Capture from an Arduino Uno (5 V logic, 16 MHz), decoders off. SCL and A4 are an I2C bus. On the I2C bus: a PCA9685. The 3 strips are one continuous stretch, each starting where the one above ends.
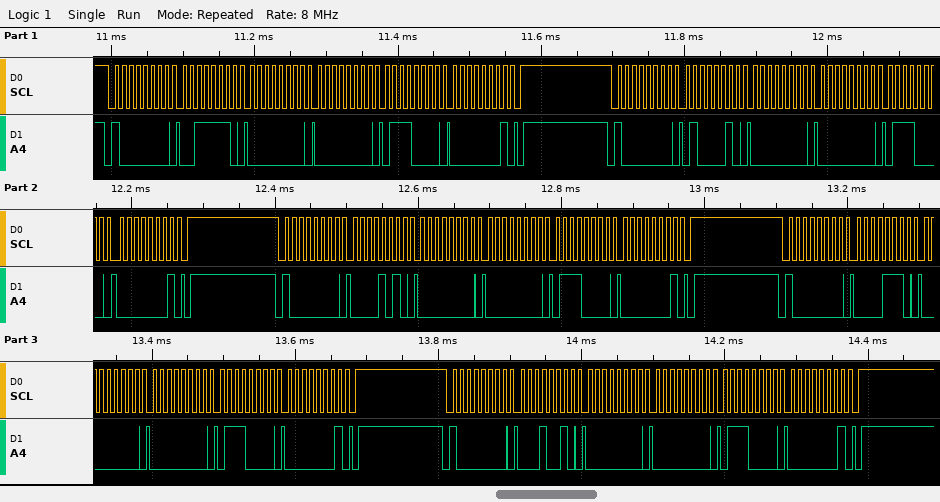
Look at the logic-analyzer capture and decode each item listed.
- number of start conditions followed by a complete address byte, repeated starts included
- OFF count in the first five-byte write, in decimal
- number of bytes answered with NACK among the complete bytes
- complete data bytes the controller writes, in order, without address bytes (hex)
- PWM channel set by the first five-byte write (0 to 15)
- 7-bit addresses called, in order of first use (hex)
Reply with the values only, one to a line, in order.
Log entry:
5
368
0
3E 00 00 70 01 42 00 00 70 01 0A 00 00 70 01 0E 00 00 70 01 12 00 00 70 01
14
0x40
